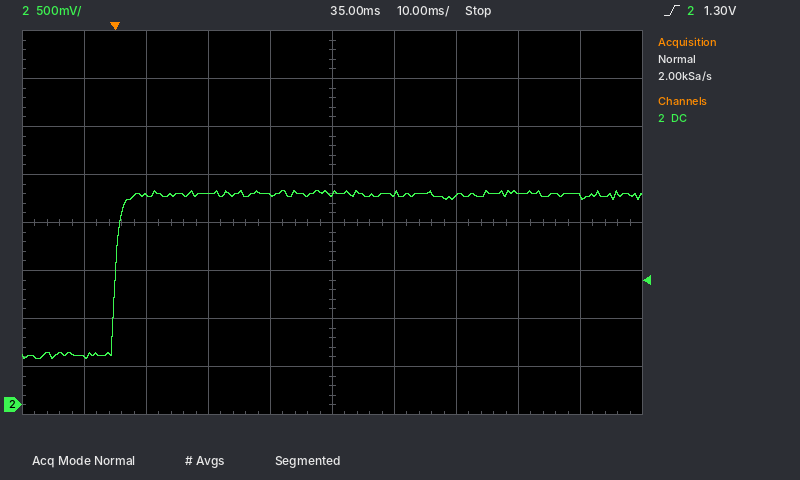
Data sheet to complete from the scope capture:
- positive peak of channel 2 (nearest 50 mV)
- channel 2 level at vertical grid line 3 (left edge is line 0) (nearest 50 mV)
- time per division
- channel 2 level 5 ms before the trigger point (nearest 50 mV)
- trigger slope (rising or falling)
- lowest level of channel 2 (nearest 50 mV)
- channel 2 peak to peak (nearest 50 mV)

2.25 V
2.20 V
10 ms
500 mV
rising
500 mV
1.75 V
